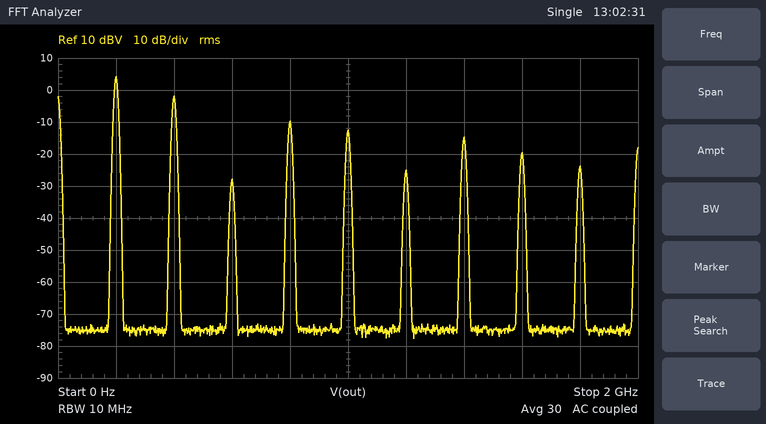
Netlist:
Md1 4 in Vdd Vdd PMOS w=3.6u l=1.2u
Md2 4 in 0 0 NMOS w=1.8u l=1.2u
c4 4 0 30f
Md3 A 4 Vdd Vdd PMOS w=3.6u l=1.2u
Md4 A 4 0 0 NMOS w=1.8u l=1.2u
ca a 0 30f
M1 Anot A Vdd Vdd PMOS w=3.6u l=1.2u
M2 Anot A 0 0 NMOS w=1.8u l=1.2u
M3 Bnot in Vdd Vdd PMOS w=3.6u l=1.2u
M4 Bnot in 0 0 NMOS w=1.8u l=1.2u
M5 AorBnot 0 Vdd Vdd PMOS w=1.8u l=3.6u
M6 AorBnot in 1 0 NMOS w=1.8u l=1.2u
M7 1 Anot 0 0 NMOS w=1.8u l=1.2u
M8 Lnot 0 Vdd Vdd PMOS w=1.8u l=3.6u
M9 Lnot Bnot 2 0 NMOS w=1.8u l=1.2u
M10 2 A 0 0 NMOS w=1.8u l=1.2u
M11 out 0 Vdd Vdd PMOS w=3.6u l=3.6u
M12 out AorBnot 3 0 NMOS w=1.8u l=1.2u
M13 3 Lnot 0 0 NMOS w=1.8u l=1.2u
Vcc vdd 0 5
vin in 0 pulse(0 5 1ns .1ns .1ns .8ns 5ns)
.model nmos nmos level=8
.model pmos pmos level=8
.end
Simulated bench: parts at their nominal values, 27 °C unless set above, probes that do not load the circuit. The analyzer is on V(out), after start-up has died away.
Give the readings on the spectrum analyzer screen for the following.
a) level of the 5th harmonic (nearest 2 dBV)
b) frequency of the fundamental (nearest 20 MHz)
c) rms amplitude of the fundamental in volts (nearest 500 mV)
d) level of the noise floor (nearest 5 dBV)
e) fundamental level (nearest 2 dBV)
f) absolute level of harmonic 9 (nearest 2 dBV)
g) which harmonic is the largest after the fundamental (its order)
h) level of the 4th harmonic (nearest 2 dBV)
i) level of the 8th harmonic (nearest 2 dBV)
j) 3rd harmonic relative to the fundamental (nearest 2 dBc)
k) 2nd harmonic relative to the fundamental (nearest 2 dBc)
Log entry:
-12 dBV
200 MHz
1.5 V
-75 dBV
4 dBV
-24 dBV
2
-10 dBV
-20 dBV
-32 dBc
-6 dBc
